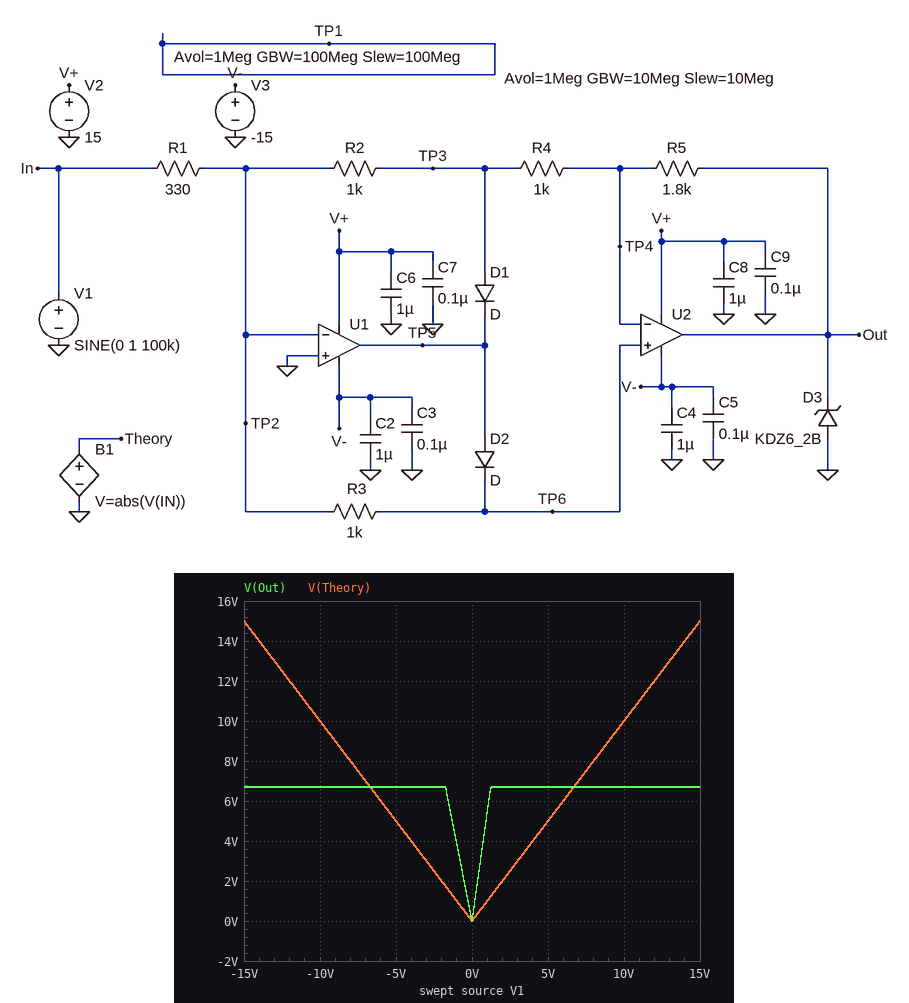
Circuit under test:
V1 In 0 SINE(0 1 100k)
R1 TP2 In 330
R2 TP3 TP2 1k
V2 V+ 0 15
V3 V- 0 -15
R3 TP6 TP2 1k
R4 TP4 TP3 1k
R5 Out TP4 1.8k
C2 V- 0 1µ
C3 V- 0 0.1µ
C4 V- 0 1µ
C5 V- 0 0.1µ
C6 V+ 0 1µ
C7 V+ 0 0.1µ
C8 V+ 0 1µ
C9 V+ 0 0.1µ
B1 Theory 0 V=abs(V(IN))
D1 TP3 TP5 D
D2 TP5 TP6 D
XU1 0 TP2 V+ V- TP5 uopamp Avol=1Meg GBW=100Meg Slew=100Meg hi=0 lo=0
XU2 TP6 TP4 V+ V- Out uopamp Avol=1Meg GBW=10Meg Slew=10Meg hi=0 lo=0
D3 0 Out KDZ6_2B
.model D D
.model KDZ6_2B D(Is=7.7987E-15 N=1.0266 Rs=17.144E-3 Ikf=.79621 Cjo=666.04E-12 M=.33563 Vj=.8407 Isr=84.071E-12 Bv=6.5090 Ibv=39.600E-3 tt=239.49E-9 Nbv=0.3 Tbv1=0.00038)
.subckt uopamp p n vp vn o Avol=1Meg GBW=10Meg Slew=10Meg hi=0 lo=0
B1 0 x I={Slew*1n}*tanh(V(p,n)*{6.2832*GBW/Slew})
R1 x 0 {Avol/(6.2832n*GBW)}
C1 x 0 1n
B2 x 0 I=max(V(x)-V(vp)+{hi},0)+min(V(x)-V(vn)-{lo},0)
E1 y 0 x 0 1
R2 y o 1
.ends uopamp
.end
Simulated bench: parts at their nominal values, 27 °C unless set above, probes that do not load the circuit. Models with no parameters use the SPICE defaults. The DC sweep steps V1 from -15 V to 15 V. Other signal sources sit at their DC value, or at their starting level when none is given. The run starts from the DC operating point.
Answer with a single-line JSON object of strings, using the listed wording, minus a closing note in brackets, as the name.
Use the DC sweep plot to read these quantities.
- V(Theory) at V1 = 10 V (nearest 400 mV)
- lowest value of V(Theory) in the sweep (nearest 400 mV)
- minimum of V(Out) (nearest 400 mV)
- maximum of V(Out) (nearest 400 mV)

{"V(Theory) at V1 = 10 V": "10.0 V", "lowest value of V(Theory) in the sweep": "0 V", "minimum of V(Out)": "0 V", "maximum of V(Out)": "6.8 V"}
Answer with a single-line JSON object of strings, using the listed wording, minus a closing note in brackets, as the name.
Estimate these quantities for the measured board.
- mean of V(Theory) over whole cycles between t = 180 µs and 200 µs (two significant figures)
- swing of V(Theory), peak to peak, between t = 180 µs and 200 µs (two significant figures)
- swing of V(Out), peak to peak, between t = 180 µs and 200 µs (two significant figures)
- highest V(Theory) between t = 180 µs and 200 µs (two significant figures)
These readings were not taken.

{"mean of V(Theory) over whole cycles between t = 180 µs and 200 µs": "640 mV", "swing of V(Theory), peak to peak, between t = 180 µs and 200 µs": "1.0 V", "swing of V(Out), peak to peak, between t = 180 µs and 200 µs": "5.5 V", "highest V(Theory) between t = 180 µs and 200 µs": "1.0 V"}
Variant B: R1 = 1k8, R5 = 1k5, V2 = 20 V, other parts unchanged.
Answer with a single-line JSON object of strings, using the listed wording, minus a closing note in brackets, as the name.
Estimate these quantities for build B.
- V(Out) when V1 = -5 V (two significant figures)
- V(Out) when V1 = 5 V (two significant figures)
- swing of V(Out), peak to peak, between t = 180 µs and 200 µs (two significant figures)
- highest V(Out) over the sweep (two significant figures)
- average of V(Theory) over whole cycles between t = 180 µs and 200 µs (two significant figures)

{"V(Out) when V1 = -5 V": "3.2 V", "V(Out) when V1 = 5 V": "4.2 V", "swing of V(Out), peak to peak, between t = 180 µs and 200 µs": "860 mV", "highest V(Out) over the sweep": "6.8 V", "average of V(Theory) over whole cycles between t = 180 µs and 200 µs": "640 mV"}
